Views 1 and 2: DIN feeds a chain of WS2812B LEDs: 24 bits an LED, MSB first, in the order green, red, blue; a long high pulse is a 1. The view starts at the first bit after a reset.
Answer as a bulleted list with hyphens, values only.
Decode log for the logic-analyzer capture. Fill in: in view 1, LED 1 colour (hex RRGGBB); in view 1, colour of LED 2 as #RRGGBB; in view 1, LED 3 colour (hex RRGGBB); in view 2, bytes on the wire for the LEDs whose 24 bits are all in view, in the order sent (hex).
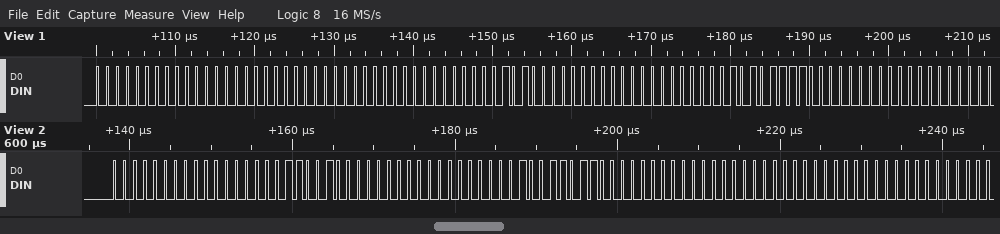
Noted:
- #000000
- #000050
- #0000AF
- 00 00 64 00 00 9B 00 00 00
